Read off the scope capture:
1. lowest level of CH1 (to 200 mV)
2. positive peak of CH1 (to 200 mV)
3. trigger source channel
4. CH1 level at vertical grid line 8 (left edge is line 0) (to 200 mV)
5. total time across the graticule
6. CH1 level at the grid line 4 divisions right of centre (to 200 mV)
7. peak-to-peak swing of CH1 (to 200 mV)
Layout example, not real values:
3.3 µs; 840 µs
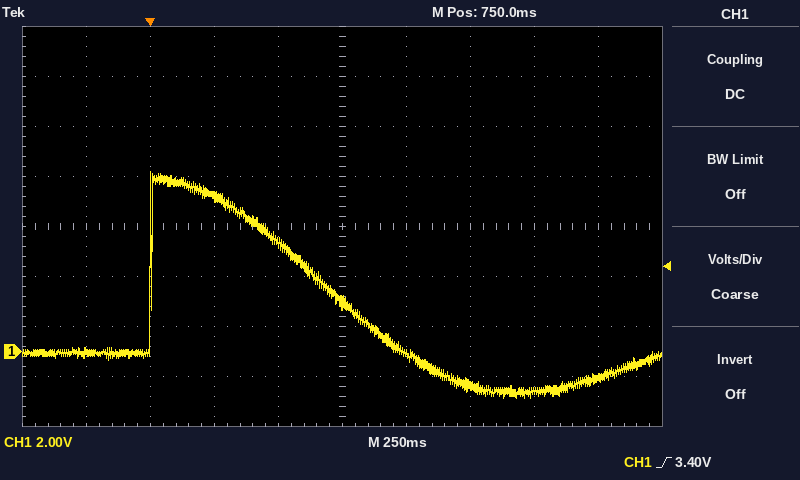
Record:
-1.8 V; 7.2 V; CH1; -1.6 V; 2.5 s; -1.0 V; 9.0 V
